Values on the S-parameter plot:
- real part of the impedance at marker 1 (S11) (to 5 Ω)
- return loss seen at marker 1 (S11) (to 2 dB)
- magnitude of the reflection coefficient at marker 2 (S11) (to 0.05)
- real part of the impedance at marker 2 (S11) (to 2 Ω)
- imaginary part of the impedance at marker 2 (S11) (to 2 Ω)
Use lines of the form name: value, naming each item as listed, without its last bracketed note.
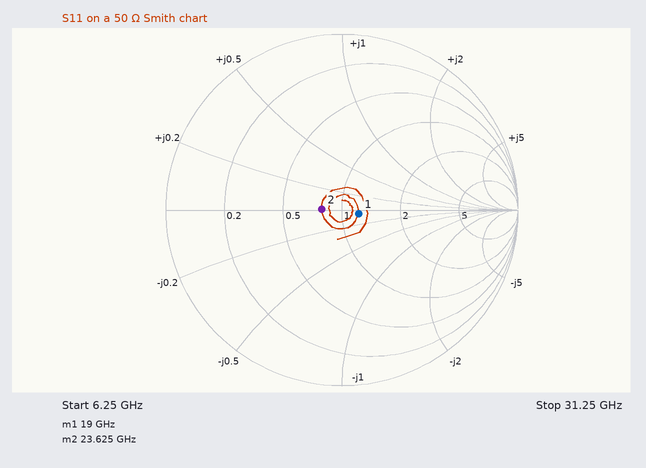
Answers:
real part of the impedance at marker 1 (S11): 60 Ω
return loss seen at marker 1 (S11): 20 dB
magnitude of the reflection coefficient at marker 2 (S11): 0.10
real part of the impedance at marker 2 (S11): 40 Ω
imaginary part of the impedance at marker 2 (S11): 0 Ω
